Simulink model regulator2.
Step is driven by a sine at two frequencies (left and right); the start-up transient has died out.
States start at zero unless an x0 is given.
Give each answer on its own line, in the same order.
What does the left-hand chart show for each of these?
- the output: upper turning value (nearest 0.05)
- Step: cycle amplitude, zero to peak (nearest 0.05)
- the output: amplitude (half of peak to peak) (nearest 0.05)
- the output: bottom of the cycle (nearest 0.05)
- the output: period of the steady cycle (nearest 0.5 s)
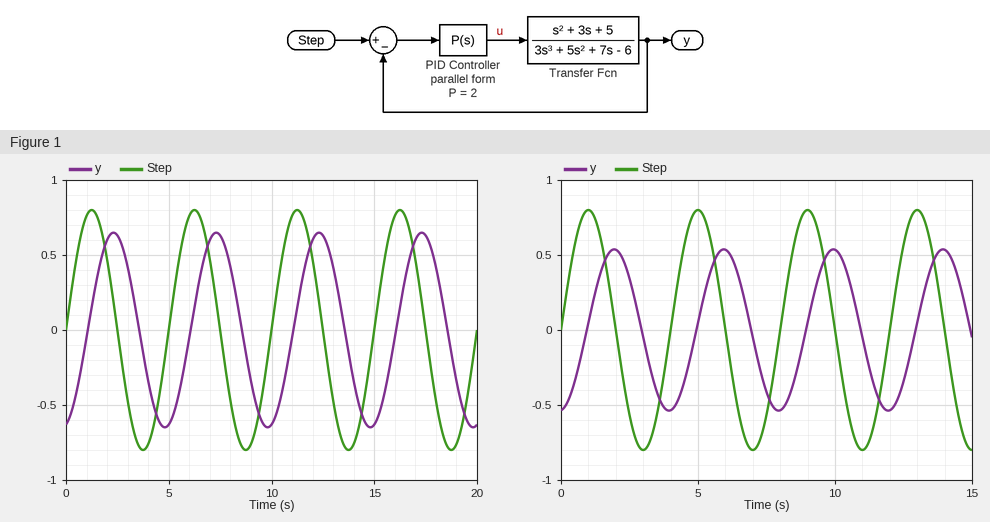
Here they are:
0.65
0.80
0.65
-0.65
5.0 s
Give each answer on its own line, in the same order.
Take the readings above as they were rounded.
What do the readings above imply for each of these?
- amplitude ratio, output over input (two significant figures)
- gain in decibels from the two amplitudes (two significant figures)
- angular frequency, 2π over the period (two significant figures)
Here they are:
0.81
-1.8 dB
1.3 rad/s
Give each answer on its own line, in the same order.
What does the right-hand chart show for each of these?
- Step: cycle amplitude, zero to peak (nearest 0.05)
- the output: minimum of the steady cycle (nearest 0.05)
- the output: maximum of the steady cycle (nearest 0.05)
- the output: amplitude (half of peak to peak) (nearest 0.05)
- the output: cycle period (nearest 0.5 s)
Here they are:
0.80
-0.55
0.55
0.55
4.0 s
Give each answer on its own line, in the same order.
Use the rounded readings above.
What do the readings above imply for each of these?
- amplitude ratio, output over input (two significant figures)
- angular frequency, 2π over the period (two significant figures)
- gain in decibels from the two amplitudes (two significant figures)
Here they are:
0.69
1.6 rad/s
-3.3 dB
